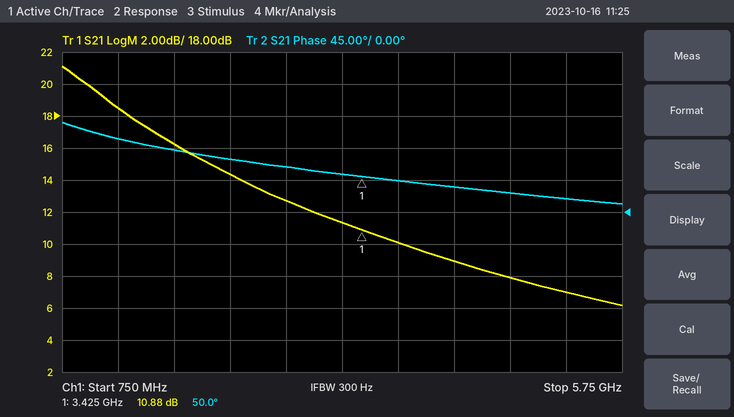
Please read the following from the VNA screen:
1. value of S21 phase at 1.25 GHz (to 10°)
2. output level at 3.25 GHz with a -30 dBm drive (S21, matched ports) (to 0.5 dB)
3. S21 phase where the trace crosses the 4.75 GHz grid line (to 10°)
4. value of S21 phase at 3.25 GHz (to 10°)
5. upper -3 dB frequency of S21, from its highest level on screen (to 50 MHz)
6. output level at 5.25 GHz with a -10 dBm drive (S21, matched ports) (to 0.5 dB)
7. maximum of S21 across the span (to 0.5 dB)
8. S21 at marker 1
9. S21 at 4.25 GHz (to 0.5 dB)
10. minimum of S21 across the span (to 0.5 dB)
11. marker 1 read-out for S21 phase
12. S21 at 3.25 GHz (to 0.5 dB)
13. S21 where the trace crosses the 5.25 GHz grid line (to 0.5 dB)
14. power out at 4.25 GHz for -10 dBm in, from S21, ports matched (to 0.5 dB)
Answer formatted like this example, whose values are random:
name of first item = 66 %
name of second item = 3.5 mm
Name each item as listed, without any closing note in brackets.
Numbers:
value of S21 phase at 1.25 GHz = 100°
output level at 3.25 GHz with a -30 dBm drive (S21, matched ports) = -18.5 dBm
S21 phase where the trace crosses the 4.75 GHz grid line = 30°
value of S21 phase at 3.25 GHz = 50°
upper -3 dB frequency of S21, from its highest level on screen = 1.35 GHz
output level at 5.25 GHz with a -10 dBm drive (S21, matched ports) = -3.0 dBm
maximum of S21 across the span = 21.0 dB
S21 at marker 1 = 10.88 dB
S21 at 4.25 GHz = 9.0 dB
minimum of S21 across the span = 6.0 dB
marker 1 read-out for S21 phase = 50.0°
S21 at 3.25 GHz = 11.5 dB
S21 where the trace crosses the 5.25 GHz grid line = 7.0 dB
power out at 4.25 GHz for -10 dBm in, from S21, ports matched = -1.0 dBm
